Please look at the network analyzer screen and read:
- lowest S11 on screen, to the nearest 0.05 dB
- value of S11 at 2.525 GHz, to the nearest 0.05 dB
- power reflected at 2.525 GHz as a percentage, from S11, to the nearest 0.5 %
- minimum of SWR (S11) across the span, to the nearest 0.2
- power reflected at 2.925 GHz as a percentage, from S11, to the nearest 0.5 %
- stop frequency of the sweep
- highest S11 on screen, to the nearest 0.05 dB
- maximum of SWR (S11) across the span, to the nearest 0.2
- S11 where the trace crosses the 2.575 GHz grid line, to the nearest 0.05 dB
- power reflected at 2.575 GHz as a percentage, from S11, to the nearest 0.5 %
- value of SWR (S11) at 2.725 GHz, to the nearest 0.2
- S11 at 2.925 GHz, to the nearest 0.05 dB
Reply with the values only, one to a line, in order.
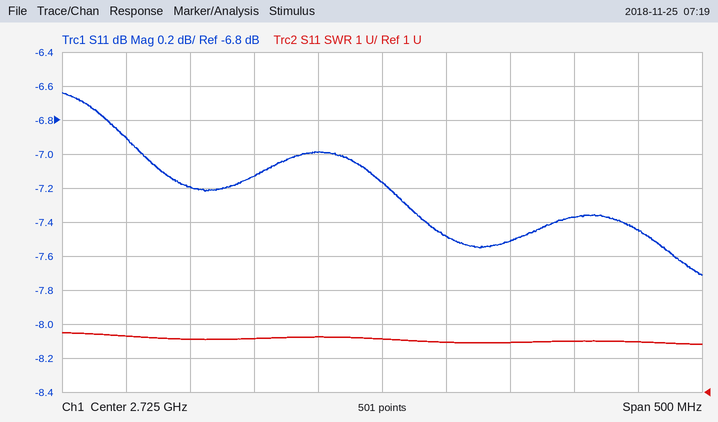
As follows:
-7.70 dB
-6.90 dB
20.5 %
2.4
18.0 %
2.975 GHz
-6.65 dB
2.8
-7.20 dB
19.0 %
2.6
-7.45 dB
